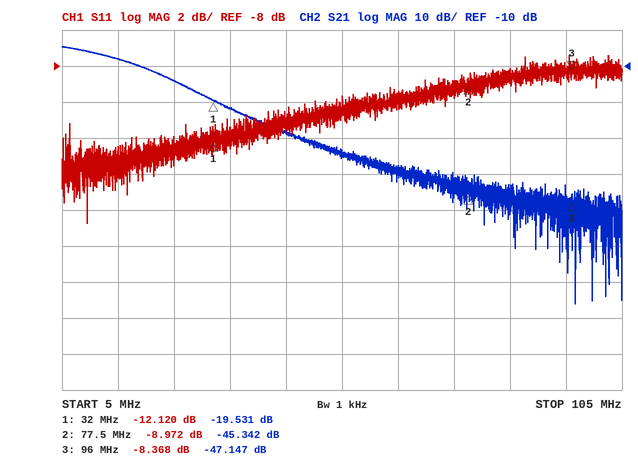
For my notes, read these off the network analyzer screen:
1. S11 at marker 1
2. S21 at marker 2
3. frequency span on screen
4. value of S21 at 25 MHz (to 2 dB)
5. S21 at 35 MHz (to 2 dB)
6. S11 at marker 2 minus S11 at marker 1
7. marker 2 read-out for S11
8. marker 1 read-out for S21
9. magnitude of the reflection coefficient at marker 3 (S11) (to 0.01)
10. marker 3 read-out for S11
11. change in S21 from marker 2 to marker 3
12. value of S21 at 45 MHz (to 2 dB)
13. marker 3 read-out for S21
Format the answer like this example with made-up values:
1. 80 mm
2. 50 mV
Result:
1. -12.120 dB
2. -45.342 dB
3. 100 MHz
4. -14 dB
5. -22 dB
6. 3.148 dB
7. -8.972 dB
8. -19.531 dB
9. 0.38
10. -8.368 dB
11. -1.805 dB
12. -28 dB
13. -47.147 dB
